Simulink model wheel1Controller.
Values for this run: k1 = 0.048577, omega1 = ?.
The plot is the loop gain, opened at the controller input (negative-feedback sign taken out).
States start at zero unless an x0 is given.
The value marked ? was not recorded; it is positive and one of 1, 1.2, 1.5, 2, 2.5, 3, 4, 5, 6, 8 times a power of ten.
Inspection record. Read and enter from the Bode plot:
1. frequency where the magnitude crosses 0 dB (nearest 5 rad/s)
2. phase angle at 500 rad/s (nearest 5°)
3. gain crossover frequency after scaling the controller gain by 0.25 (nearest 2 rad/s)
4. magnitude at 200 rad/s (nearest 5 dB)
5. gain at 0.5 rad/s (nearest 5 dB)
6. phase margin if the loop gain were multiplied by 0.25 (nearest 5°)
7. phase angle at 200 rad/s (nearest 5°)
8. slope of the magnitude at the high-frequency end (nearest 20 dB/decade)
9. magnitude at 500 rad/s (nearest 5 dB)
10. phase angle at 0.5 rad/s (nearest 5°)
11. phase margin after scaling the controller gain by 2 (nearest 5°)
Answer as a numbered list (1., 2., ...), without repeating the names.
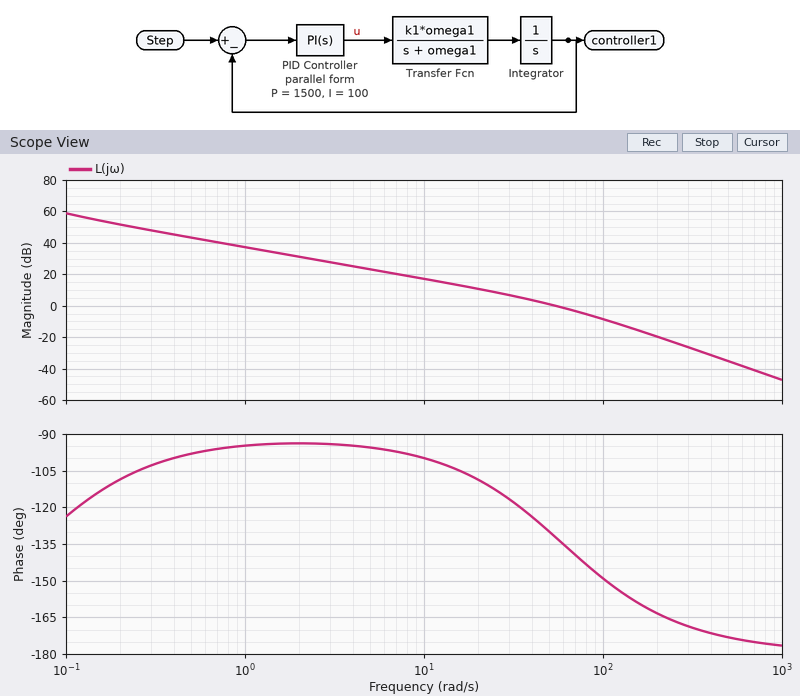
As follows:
1. 55 rad/s
2. -175°
3. 18 rad/s
4. -20 dB
5. 45 dB
6. 75°
7. -165°
8. -40 dB/decade
9. -35 dB
10. -100°
11. 35°
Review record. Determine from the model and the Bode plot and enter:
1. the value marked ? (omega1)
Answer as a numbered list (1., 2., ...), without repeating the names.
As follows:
1. 60
